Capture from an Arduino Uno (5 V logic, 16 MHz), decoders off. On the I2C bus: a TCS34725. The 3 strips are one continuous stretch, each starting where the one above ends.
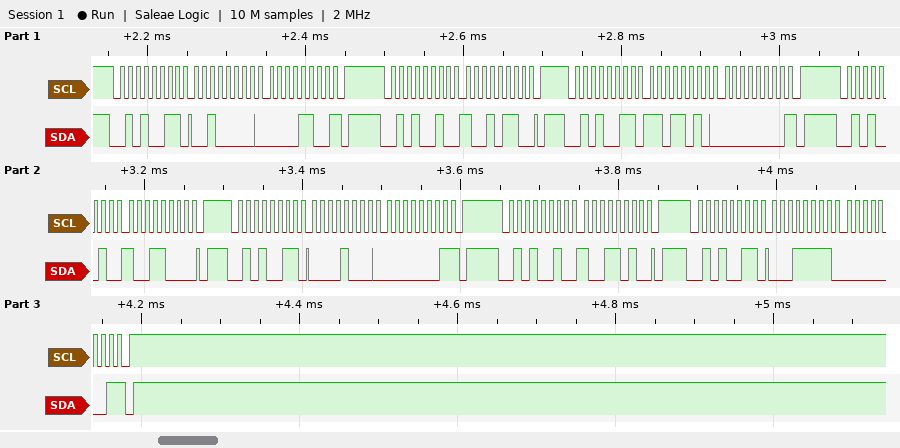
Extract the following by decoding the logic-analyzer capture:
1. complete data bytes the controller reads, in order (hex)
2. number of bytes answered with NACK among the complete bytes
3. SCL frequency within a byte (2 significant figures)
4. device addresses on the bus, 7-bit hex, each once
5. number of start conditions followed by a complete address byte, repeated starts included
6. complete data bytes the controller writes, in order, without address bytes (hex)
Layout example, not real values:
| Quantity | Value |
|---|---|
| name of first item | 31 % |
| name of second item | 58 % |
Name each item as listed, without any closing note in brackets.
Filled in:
| Quantity | Value |
|---|---|
| complete data bytes the controller reads, in order | 20 0C DA 00 08 01 1F 01 |
| number of bytes answered with NACK among the complete bytes | 4 |
| SCL frequency within a byte | 100 kHz |
| device addresses on the bus, 7-bit hex, each once | 0x29 |
| number of start conditions followed by a complete address byte, repeated starts included | 7 |
| complete data bytes the controller writes, in order, without address bytes | 96 98 9A |
